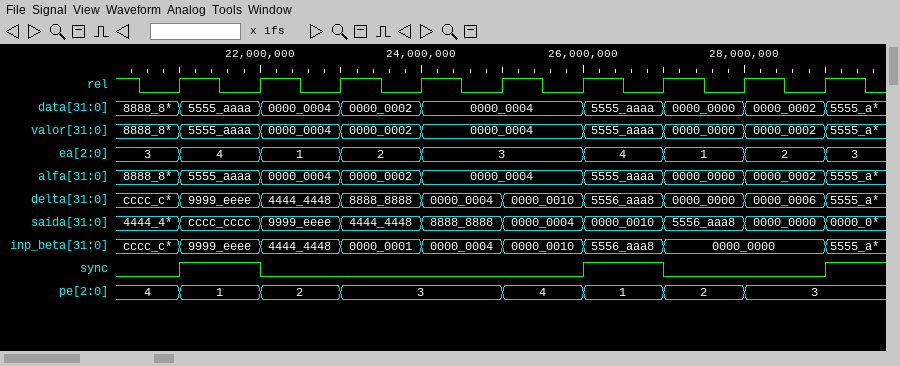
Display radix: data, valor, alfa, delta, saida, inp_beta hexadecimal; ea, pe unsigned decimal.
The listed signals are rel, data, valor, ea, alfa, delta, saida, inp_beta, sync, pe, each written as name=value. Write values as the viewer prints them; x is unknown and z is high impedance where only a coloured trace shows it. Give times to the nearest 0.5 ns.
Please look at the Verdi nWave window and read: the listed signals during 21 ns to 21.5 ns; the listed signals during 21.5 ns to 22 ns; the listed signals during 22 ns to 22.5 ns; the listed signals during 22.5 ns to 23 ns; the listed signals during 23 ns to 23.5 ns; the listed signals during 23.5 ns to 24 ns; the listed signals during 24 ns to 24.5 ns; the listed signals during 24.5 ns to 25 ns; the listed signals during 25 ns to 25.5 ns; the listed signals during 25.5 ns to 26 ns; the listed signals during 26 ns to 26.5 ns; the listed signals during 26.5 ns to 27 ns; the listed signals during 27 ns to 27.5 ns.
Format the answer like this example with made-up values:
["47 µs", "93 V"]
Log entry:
["rel=1, data=5555_aaaa, valor=5555_aaaa, ea=4, alfa=5555_aaaa, delta=9999_eeee, saida=cccc_cccc, inp_beta=9999_eeee, sync=1, pe=1", "rel=0, data=5555_aaaa, valor=5555_aaaa, ea=4, alfa=5555_aaaa, delta=9999_eeee, saida=cccc_cccc, inp_beta=9999_eeee, sync=1, pe=1", "rel=1, data=0000_0004, valor=0000_0004, ea=1, alfa=0000_0004, delta=4444_4448, saida=9999_eeee, inp_beta=4444_4448, sync=0, pe=2", "rel=0, data=0000_0004, valor=0000_0004, ea=1, alfa=0000_0004, delta=4444_4448, saida=9999_eeee, inp_beta=4444_4448, sync=0, pe=2", "rel=1, data=0000_0002, valor=0000_0002, ea=2, alfa=0000_0002, delta=8888_8888, saida=4444_4448, inp_beta=0000_0001, sync=0, pe=3", "rel=0, data=0000_0002, valor=0000_0002, ea=2, alfa=0000_0002, delta=8888_8888, saida=4444_4448, inp_beta=0000_0001, sync=0, pe=3", "rel=1, data=0000_0004, valor=0000_0004, ea=3, alfa=0000_0004, delta=0000_0004, saida=8888_8888, inp_beta=0000_0004, sync=0, pe=3", "rel=0, data=0000_0004, valor=0000_0004, ea=3, alfa=0000_0004, delta=0000_0004, saida=8888_8888, inp_beta=0000_0004, sync=0, pe=3", "rel=1, data=0000_0004, valor=0000_0004, ea=3, alfa=0000_0004, delta=0000_0010, saida=0000_0004, inp_beta=0000_0010, sync=0, pe=4", "rel=0, data=0000_0004, valor=0000_0004, ea=3, alfa=0000_0004, delta=0000_0010, saida=0000_0004, inp_beta=0000_0010, sync=0, pe=4", "rel=1, data=5555_aaaa, valor=5555_aaaa, ea=4, alfa=5555_aaaa, delta=5556_aaa8, saida=0000_0010, inp_beta=5556_aaa8, sync=1, pe=1", "rel=0, data=5555_aaaa, valor=5555_aaaa, ea=4, alfa=5555_aaaa, delta=5556_aaa8, saida=0000_0010, inp_beta=5556_aaa8, sync=1, pe=1", "rel=1, data=0000_0000, valor=0000_0000, ea=1, alfa=0000_0000, delta=0000_0000, saida=5556_aaa8, inp_beta=0000_0000, sync=0, pe=2"]
